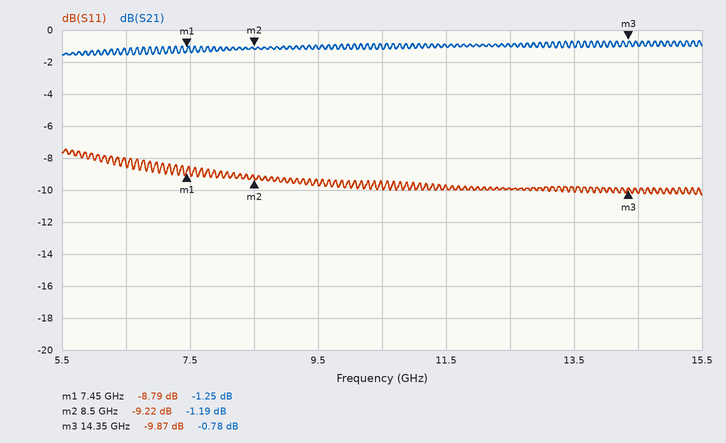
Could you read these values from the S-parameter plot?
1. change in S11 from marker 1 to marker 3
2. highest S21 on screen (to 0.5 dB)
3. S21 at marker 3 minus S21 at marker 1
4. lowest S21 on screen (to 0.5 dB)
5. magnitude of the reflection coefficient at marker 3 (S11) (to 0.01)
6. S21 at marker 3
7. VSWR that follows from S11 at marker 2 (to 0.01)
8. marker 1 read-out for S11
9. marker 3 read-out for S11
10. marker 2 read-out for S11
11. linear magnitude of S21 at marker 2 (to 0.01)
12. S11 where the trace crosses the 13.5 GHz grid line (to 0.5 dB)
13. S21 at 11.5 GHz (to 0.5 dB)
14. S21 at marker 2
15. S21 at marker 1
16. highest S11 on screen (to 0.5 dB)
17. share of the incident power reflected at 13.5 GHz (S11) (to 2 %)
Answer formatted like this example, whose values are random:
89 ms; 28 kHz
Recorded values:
-1.08 dB; -0.5 dB; 0.47 dB; -1.5 dB; 0.32; -0.78 dB; 2.06; -8.79 dB; -9.87 dB; -9.22 dB; 0.87; -10.0 dB; -1.0 dB; -1.19 dB; -1.25 dB; -7.5 dB; 10 %
